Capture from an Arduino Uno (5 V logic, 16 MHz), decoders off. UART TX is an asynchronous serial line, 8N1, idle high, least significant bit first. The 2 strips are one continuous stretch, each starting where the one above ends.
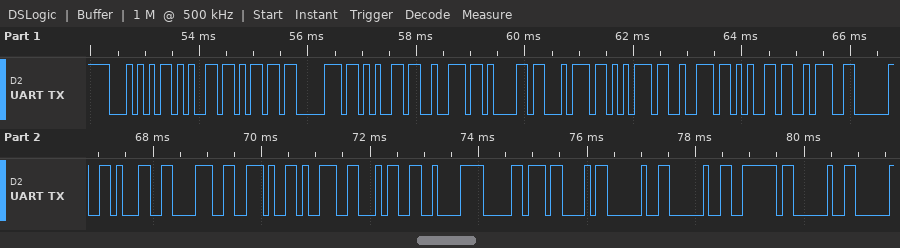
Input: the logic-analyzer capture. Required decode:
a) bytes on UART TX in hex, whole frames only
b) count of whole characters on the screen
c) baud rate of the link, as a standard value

54 65 6D 70 65 72 61 74 75 72 65 3A 20 31 38 2E 39 34 C2 B0 43 20 20 7E 20
25
9600 baud
